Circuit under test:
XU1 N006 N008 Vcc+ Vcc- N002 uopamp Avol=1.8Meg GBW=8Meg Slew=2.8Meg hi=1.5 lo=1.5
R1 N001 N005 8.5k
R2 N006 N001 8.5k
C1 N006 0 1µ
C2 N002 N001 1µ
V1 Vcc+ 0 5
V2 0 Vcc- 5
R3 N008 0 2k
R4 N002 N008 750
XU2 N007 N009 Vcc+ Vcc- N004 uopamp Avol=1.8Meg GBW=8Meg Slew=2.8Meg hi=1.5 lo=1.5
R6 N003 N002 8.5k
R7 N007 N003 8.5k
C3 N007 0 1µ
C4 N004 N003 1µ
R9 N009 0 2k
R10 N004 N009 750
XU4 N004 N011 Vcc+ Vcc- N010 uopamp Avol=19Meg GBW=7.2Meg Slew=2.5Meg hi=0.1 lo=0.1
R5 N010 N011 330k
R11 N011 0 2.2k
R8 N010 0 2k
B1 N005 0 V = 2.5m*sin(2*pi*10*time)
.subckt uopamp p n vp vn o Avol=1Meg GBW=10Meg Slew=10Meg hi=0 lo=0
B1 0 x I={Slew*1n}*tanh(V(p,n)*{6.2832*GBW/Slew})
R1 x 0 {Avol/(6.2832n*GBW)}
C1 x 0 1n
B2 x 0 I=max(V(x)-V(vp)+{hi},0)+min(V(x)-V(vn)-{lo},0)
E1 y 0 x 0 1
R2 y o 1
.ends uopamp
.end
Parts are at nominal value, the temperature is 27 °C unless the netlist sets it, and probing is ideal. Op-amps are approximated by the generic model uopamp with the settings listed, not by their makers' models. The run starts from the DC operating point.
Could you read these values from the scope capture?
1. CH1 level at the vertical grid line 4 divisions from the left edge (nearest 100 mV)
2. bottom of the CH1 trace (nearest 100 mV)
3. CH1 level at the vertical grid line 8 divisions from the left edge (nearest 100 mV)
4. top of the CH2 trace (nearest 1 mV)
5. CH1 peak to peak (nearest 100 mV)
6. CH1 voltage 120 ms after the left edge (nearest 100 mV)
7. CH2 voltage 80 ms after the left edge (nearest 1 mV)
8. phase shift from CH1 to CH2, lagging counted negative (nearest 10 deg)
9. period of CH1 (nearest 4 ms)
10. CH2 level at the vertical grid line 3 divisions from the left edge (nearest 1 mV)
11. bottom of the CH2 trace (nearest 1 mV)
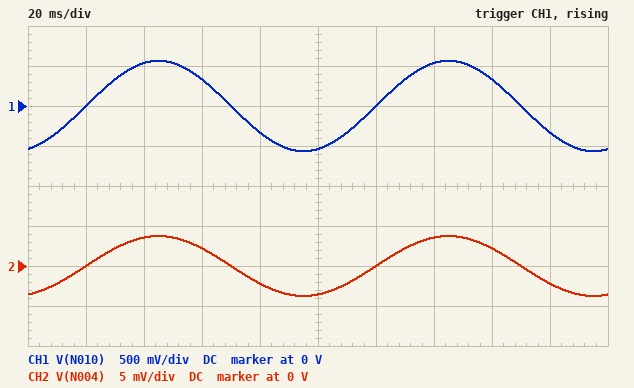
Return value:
-300 mV
-600 mV
300 mV
4 mV
1.1 V
0 V
-2 mV
0 deg
100 ms
2 mV
-4 mV
